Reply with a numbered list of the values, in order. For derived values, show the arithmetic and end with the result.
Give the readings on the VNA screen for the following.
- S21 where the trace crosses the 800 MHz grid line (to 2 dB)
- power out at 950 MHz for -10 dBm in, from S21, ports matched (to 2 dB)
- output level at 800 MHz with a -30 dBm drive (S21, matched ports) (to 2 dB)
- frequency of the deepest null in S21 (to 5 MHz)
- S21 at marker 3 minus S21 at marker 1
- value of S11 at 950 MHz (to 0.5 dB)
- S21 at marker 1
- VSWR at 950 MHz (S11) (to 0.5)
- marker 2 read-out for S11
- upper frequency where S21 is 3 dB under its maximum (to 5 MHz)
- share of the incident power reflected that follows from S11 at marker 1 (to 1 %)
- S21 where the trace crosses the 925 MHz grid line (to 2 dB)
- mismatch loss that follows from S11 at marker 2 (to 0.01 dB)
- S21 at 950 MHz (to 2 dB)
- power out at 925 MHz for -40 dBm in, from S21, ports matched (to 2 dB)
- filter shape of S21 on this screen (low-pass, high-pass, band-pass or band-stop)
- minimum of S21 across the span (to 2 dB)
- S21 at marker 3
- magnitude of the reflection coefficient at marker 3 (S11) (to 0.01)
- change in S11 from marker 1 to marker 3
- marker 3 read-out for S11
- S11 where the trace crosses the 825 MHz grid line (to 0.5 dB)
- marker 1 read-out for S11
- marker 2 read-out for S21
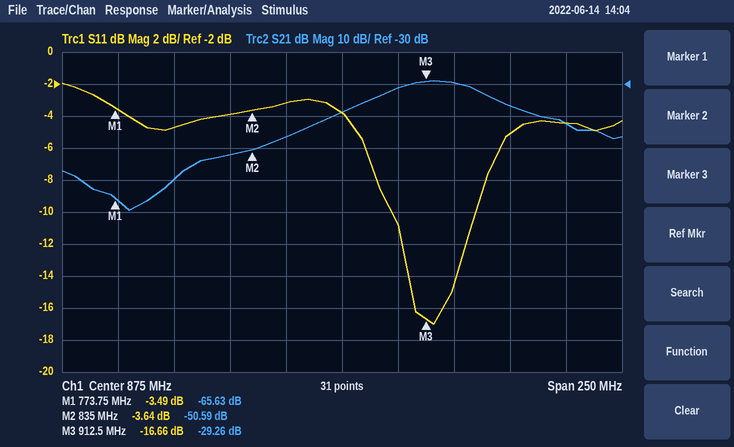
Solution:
1. -60 dB
2. -10 dBm + (-36 dB) = -46 dBm
3. -30 dBm + (-60 dB) = -90 dBm
4. 780 MHz
5. -29.26 − (-65.63) = 36.37 dB
6. -5.0 dB
7. -65.63 dB
8. |Γ| = 10^(-5/20) = 0.5623; VSWR = (1 + 0.5623)/(1 − 0.5623) ≈ 3.57, so 3.5 to the nearest 0.5
9. -3.64 dB
10. 935 MHz
11. 10^(-3.49/10) ≈ 45 %
12. -30 dB
13. −10 log10(1 − 10^(-3.64/10)) ≈ 2.46 dB
14. -36 dB
15. -40 dBm + (-30 dB) = -70 dBm
16. band-pass
17. -70 dB
18. -29.26 dB
19. 10^(-16.66/20) ≈ 0.15
20. -16.66 − (-3.49) = -13.17 dB
21. -16.66 dB
22. -4.0 dB
23. -3.49 dB
24. -50.59 dB
